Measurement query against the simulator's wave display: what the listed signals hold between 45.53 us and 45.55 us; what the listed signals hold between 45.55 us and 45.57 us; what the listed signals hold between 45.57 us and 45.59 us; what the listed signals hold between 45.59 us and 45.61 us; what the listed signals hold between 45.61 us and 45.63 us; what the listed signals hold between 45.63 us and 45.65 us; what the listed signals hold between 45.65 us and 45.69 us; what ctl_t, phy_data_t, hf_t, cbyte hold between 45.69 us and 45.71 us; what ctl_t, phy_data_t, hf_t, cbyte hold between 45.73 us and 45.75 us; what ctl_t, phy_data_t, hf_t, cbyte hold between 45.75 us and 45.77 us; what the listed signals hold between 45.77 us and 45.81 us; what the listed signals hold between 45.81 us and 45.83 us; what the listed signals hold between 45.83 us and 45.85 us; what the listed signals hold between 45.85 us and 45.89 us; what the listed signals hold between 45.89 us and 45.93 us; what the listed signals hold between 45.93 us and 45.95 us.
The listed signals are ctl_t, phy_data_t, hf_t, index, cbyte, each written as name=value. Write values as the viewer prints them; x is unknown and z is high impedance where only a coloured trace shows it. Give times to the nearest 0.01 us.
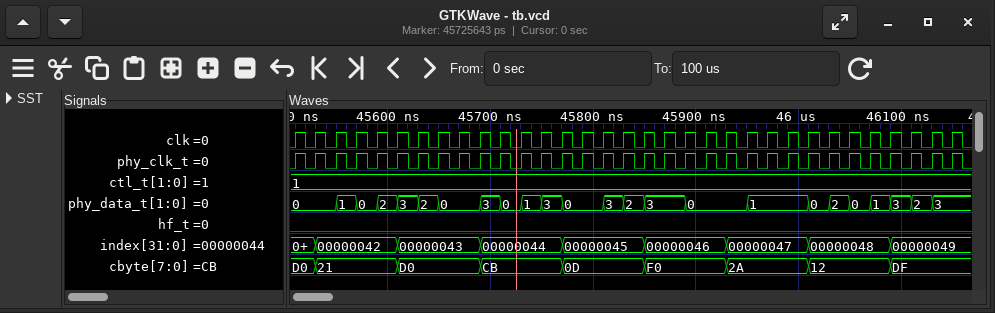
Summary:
ctl_t=1, phy_data_t=0, hf_t=0, index=00000042, cbyte=21
ctl_t=1, phy_data_t=1, hf_t=0, index=00000042, cbyte=21
ctl_t=1, phy_data_t=0, hf_t=0, index=00000042, cbyte=21
ctl_t=1, phy_data_t=2, hf_t=0, index=00000042, cbyte=21
ctl_t=1, phy_data_t=3, hf_t=0, index=00000043, cbyte=D0
ctl_t=1, phy_data_t=2, hf_t=0, index=00000043, cbyte=D0
ctl_t=1, phy_data_t=0, hf_t=0, index=00000043, cbyte=D0
ctl_t=1, phy_data_t=3, hf_t=0, cbyte=CB
ctl_t=1, phy_data_t=1, hf_t=0, cbyte=CB
ctl_t=1, phy_data_t=3, hf_t=0, cbyte=CB
ctl_t=1, phy_data_t=0, hf_t=0, index=00000045, cbyte=0D
ctl_t=1, phy_data_t=3, hf_t=0, index=00000045, cbyte=0D
ctl_t=1, phy_data_t=2, hf_t=0, index=00000045, cbyte=0D
ctl_t=1, phy_data_t=3, hf_t=0, index=00000046, cbyte=F0
ctl_t=1, phy_data_t=0, hf_t=0, index=00000046, cbyte=F0
ctl_t=1, phy_data_t=0, hf_t=0, index=00000047, cbyte=2A
